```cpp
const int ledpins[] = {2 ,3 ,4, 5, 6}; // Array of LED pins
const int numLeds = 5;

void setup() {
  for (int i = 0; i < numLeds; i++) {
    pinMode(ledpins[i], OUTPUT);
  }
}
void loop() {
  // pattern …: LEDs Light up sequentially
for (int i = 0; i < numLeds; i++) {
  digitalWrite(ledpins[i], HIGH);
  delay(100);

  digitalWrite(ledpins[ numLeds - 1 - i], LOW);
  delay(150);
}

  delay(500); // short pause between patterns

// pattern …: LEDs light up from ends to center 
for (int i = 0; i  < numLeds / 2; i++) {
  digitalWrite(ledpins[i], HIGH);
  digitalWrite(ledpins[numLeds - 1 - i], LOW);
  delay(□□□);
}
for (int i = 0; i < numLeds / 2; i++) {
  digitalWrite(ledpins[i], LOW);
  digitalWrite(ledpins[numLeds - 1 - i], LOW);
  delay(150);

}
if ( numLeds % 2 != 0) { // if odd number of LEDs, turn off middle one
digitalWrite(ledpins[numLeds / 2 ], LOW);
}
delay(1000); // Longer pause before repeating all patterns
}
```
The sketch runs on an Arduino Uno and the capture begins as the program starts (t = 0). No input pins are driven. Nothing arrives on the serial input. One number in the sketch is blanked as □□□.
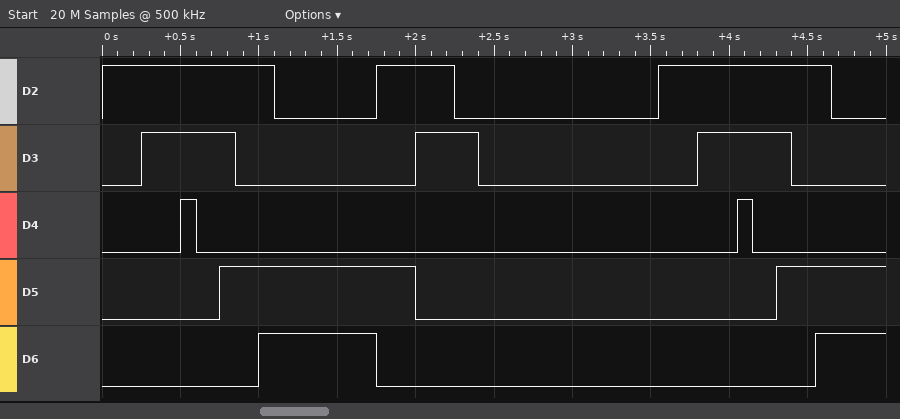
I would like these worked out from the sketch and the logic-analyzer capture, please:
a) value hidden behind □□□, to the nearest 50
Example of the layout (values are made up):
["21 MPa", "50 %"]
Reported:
["250"]
